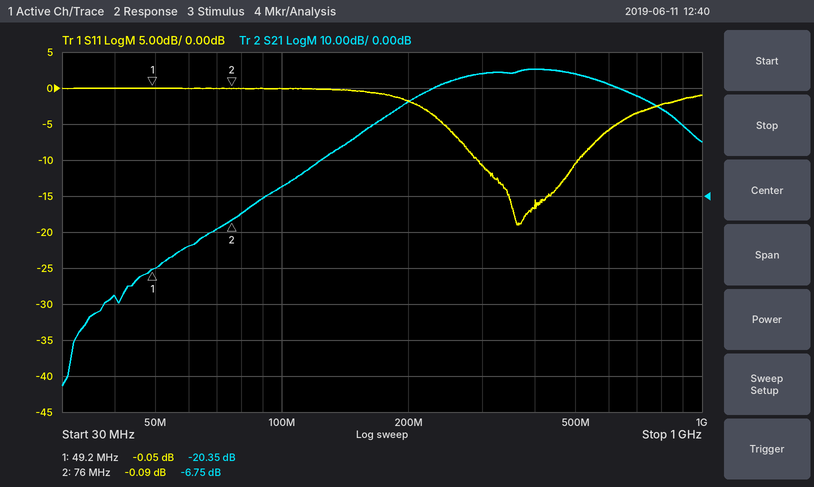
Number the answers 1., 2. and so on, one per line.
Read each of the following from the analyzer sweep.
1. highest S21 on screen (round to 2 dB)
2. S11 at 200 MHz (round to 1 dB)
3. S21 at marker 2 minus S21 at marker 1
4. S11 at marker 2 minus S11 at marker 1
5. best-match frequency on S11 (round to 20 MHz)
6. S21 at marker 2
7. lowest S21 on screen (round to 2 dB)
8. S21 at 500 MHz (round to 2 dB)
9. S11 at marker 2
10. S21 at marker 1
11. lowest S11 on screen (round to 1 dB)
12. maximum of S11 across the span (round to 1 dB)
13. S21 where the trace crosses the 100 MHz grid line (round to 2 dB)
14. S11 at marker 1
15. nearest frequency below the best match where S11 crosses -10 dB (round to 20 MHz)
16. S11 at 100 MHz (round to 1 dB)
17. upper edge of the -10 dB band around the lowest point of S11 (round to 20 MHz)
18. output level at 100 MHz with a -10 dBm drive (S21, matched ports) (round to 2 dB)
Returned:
1. 36 dB
2. -2 dB
3. 13.60 dB
4. -0.04 dB
5. 360 MHz
6. -6.75 dB
7. -52 dB
8. 34 dB
9. -0.09 dB
10. -20.35 dB
11. -19 dB
12. 0 dB
13. 2 dB
14. -0.05 dB
15. 300 MHz
16. 0 dB
17. 500 MHz
18. -8 dBm
